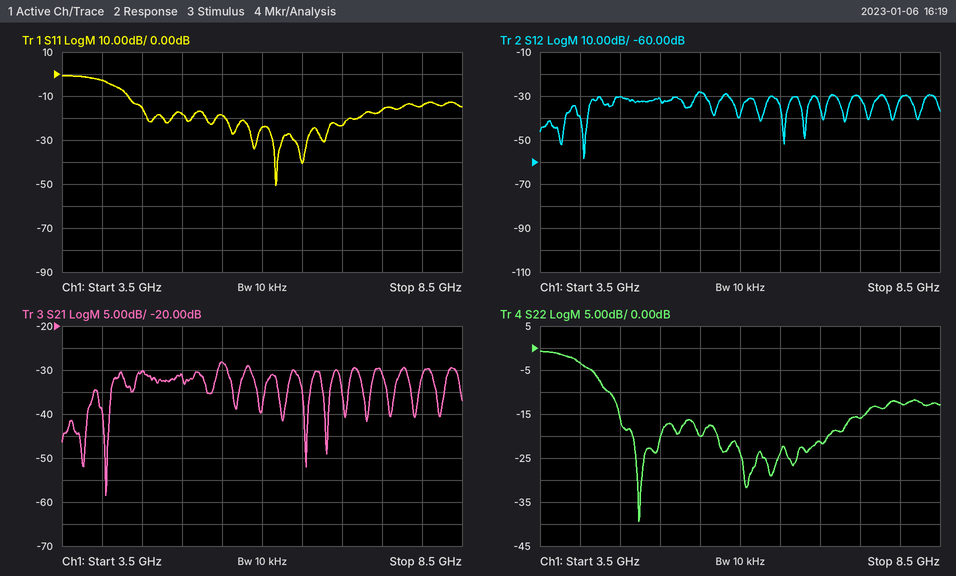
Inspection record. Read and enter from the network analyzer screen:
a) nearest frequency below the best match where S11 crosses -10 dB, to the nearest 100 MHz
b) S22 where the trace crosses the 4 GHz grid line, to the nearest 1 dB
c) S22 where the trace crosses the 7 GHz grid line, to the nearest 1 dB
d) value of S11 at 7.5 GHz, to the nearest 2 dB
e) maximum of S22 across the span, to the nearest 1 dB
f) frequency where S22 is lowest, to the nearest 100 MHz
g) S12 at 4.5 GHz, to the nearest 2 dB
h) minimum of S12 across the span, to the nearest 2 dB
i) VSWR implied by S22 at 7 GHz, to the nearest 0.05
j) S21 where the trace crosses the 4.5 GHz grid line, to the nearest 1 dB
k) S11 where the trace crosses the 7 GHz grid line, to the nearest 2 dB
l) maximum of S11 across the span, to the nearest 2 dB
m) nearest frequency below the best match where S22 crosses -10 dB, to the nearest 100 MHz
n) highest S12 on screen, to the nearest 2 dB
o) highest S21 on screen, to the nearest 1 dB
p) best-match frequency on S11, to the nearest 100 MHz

4.3 GHz
-3 dB
-21 dB
-16 dB
-1 dB
4.7 GHz
-30 dB
-58 dB
1.20
-30 dB
-24 dB
0 dB
4.4 GHz
-28 dB
-28 dB
6.2 GHz
